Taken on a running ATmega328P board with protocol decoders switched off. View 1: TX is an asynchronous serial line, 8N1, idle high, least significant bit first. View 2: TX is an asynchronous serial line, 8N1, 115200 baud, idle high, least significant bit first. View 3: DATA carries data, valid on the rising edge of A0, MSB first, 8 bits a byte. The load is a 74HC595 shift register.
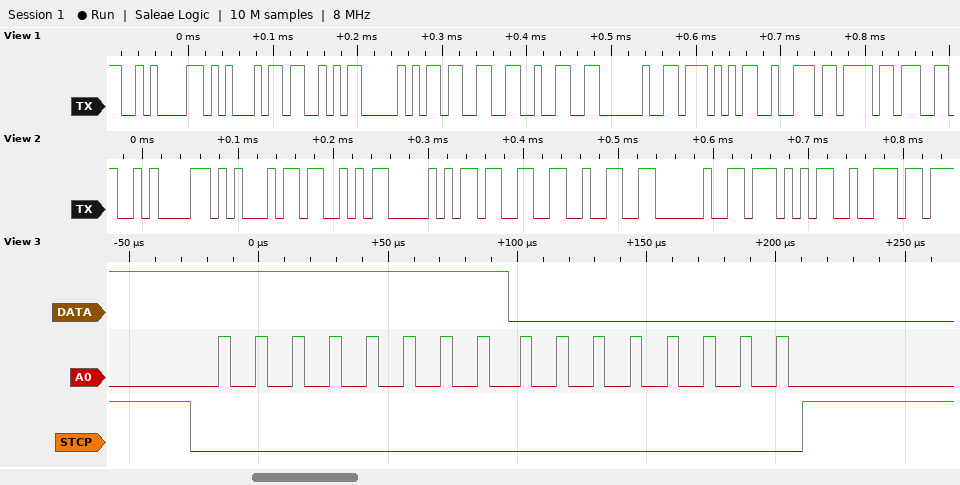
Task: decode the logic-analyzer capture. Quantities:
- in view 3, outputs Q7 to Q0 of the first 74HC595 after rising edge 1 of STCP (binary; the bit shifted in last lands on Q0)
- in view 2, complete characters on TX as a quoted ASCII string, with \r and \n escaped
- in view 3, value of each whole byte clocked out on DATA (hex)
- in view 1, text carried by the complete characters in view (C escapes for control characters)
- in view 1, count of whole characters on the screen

00000000
"\nESP32 Wr"
FF 00
"\nESP32 Wro"
10
